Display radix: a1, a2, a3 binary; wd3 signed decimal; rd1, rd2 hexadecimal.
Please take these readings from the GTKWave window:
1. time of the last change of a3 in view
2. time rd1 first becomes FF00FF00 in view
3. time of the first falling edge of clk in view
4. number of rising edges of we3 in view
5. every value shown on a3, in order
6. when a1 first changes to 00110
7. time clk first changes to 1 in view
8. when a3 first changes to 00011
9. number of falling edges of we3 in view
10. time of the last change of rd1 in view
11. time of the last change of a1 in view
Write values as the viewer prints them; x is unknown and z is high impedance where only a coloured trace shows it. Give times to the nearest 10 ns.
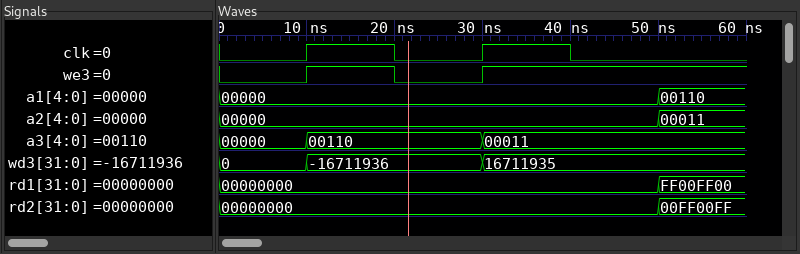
30 ns
50 ns
20 ns
2
00000, 00110, 00011
50 ns
10 ns
30 ns
1
50 ns
50 ns
